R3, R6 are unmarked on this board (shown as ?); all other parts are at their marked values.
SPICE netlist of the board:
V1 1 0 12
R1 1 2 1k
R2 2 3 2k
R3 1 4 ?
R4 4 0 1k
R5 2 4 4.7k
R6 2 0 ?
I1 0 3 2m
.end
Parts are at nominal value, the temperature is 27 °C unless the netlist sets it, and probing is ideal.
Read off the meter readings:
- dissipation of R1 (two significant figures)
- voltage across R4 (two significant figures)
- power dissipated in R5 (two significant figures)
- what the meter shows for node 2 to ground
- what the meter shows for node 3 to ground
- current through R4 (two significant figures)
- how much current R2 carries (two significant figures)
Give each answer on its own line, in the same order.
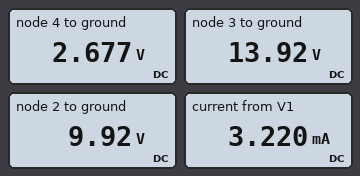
4.3 mW
2.7 V
11 mW
9.92 V
13.92 V
2.7 mA
2.0 mA
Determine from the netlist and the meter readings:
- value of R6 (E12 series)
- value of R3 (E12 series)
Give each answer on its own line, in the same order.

3.9 kΩ
8.2 kΩ
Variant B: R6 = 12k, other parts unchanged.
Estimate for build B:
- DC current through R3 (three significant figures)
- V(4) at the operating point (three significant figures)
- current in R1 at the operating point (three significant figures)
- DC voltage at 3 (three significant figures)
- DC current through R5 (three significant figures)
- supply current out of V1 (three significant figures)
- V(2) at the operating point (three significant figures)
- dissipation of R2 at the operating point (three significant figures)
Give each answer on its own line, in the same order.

1.11 mA
2.89 V
723 µA
15.3 V
1.78 mA
1.83 mA
11.3 V
8.00 mW
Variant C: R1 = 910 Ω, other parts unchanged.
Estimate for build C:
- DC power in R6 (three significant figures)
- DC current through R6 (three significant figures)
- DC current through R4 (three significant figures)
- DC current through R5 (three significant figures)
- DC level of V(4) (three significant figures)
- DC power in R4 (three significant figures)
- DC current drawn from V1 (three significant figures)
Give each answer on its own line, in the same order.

25.9 mW
2.58 mA
2.70 mA
1.56 mA
2.70 V
7.28 mW
3.28 mA
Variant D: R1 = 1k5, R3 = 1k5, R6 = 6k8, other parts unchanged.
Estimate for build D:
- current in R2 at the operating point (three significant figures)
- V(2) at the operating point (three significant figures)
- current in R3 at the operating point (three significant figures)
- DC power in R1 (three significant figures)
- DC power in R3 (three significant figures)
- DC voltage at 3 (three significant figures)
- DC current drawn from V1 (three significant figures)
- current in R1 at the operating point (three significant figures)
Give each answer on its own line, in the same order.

2.00 mA
10.9 V
4.34 mA
837 µW
28.3 mW
14.9 V
5.09 mA
747 µA
